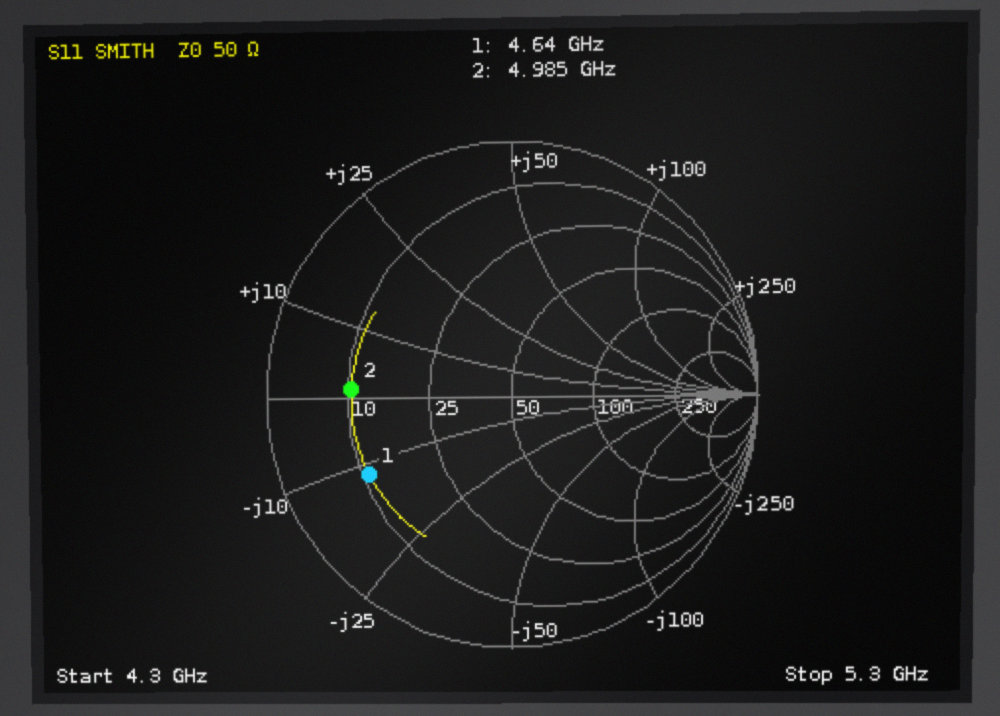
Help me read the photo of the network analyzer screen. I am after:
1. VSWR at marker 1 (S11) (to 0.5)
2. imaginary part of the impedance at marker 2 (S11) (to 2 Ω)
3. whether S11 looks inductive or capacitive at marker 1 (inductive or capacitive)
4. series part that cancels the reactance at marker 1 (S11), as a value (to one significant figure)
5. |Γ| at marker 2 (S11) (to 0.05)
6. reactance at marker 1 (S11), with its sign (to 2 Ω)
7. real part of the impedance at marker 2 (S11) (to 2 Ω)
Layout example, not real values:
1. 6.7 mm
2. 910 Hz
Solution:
1. 5.0
2. +2 Ω
3. capacitive
4. 400 pH
5. 0.65
6. -12 Ω
7. 10 Ω
